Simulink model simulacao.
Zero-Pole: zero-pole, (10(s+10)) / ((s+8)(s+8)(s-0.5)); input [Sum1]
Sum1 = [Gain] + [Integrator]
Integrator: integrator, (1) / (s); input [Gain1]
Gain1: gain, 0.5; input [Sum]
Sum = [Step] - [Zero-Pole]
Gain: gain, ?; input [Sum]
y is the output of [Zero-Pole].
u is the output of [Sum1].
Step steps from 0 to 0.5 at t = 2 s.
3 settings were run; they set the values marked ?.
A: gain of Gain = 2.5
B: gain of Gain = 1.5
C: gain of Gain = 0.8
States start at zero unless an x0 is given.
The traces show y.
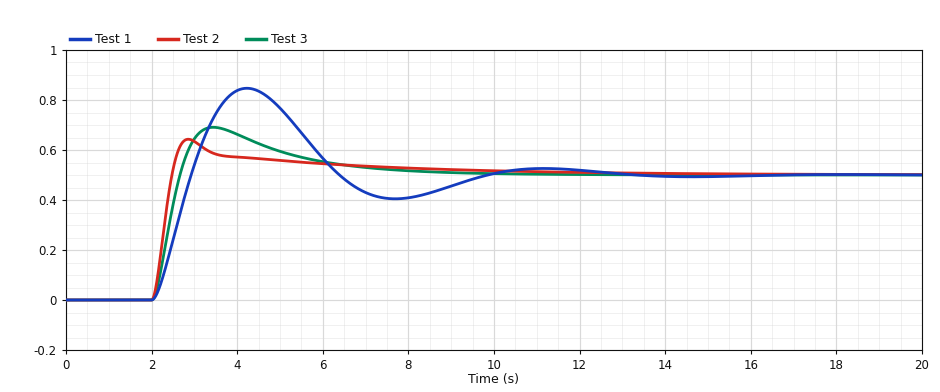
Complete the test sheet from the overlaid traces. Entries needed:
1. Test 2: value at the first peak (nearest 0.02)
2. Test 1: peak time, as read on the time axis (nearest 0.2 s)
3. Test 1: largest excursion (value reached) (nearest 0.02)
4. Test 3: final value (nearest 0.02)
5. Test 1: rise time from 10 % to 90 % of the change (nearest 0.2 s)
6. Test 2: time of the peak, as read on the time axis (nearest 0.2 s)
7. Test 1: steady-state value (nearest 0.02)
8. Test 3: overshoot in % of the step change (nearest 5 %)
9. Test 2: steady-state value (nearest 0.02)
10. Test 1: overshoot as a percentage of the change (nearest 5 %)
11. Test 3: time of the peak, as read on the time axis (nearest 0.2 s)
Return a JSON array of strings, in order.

["0.64", "4.2 s", "0.84", "0.50", "0.6 s", "2.8 s", "0.50", "40 %", "0.50", "70 %", "3.4 s"]
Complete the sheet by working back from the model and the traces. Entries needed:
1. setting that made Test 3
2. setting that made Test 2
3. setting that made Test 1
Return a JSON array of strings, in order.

["B", "A", "C"]
